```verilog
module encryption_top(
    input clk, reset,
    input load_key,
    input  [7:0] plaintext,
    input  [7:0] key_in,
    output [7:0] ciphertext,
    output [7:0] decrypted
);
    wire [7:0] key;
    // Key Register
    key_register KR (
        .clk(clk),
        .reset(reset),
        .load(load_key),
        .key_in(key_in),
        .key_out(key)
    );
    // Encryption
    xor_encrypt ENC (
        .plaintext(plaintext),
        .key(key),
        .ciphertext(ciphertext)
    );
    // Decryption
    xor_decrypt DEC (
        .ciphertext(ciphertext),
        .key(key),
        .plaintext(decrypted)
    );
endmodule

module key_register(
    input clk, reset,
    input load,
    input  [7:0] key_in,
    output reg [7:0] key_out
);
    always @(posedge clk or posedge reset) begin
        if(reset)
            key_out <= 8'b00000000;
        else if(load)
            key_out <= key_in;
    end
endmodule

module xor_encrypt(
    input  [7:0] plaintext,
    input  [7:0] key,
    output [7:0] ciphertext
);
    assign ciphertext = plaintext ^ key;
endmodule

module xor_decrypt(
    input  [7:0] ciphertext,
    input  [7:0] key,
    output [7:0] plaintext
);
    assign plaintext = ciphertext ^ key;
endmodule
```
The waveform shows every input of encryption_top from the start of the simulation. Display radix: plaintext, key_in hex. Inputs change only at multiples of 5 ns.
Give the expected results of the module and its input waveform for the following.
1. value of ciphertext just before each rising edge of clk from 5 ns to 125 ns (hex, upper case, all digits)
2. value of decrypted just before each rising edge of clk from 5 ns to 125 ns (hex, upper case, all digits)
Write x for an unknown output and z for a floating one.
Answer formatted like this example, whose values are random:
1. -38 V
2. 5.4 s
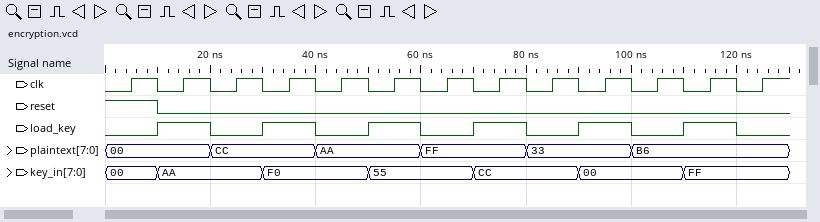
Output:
1. 00, 00, 66, 66, 5A, 5A, AA, AA, FF, FF, B6, B6, 49
2. 00, 00, CC, CC, AA, AA, FF, FF, 33, 33, B6, B6, B6
